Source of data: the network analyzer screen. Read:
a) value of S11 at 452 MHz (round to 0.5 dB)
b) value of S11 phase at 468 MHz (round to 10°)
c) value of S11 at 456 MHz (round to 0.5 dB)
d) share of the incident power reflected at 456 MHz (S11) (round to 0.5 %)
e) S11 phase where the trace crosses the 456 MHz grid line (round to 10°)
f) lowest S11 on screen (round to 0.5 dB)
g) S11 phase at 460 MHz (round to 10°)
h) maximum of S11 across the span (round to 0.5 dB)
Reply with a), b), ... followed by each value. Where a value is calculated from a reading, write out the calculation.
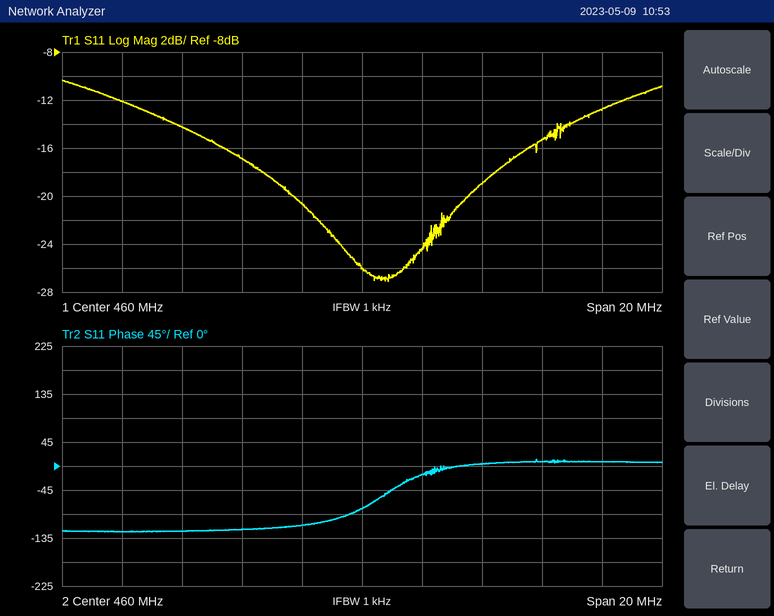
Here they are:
a) -12.0 dB
b) 10°
c) -17.0 dB
d) 10^(-17/10) ≈ 2.0 %
e) -120°
f) -27.0 dB
g) -80°
h) -10.5 dB
